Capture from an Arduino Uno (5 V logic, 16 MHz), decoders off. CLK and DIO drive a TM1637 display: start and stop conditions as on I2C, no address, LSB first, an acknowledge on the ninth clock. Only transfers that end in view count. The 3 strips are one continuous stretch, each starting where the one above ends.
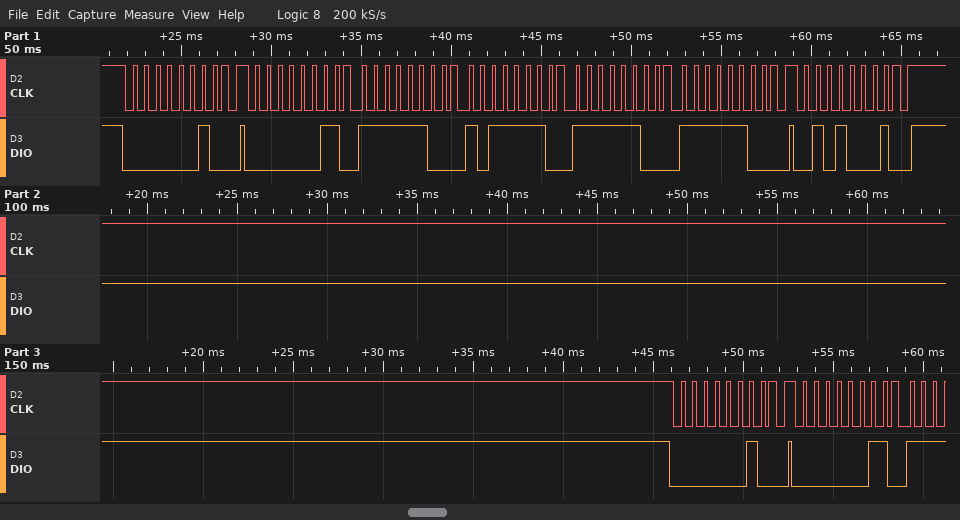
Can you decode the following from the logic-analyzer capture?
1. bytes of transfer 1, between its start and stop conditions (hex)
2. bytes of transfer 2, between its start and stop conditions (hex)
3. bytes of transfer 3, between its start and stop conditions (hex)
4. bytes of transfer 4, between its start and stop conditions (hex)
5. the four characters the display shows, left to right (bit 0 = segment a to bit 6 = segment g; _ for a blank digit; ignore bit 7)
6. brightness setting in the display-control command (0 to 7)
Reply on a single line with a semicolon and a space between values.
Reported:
40; C0 3F 7D 3F 3F; 8A; 40; 0600; 2
